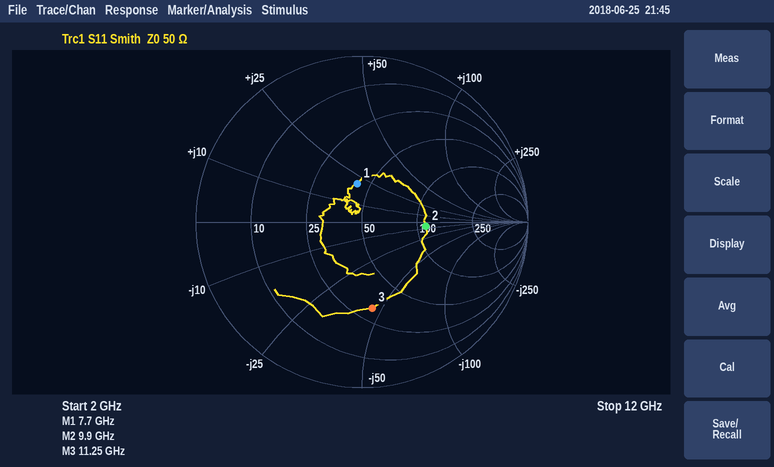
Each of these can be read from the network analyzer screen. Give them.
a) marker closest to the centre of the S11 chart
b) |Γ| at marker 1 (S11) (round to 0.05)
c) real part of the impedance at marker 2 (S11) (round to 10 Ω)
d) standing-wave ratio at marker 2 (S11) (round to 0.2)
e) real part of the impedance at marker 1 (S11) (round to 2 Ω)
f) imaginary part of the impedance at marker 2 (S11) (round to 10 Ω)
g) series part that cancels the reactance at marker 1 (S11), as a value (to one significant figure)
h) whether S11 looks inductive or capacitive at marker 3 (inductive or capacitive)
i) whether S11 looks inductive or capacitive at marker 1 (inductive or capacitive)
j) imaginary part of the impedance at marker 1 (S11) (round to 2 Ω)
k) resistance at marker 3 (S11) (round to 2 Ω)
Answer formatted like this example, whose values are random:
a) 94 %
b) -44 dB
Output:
a) marker 1
b) 0.25
c) 110 Ω
d) 2.2
e) 42 Ω
f) -10 Ω
g) 1.0 pF
h) capacitive
i) inductive
j) +20 Ω
k) 32 Ω
